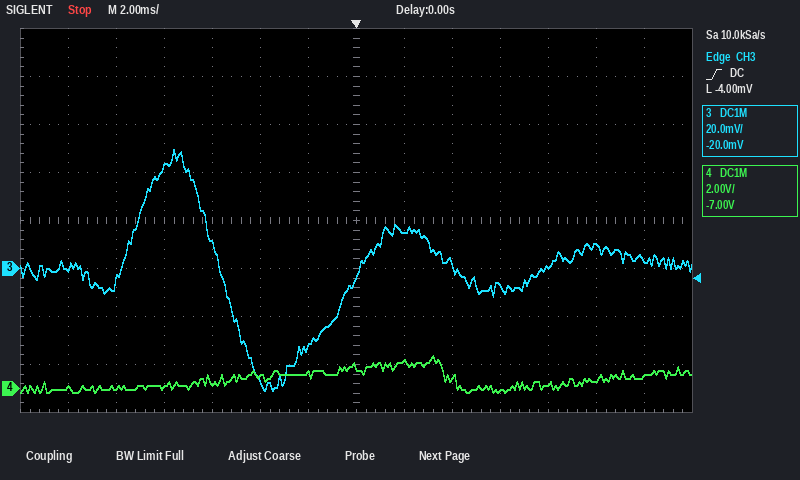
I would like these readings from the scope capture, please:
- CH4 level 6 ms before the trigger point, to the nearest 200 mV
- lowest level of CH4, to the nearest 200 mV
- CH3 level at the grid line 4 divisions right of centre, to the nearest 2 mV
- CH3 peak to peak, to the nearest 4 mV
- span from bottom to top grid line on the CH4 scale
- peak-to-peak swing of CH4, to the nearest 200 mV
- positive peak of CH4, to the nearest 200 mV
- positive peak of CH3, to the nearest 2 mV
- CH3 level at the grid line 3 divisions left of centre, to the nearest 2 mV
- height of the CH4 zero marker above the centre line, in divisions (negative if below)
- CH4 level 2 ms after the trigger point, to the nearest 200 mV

200 mV
-200 mV
0 mV
100 mV
16 V
1.6 V
1.4 V
50 mV
10 mV
-3.5 div
1.2 V
